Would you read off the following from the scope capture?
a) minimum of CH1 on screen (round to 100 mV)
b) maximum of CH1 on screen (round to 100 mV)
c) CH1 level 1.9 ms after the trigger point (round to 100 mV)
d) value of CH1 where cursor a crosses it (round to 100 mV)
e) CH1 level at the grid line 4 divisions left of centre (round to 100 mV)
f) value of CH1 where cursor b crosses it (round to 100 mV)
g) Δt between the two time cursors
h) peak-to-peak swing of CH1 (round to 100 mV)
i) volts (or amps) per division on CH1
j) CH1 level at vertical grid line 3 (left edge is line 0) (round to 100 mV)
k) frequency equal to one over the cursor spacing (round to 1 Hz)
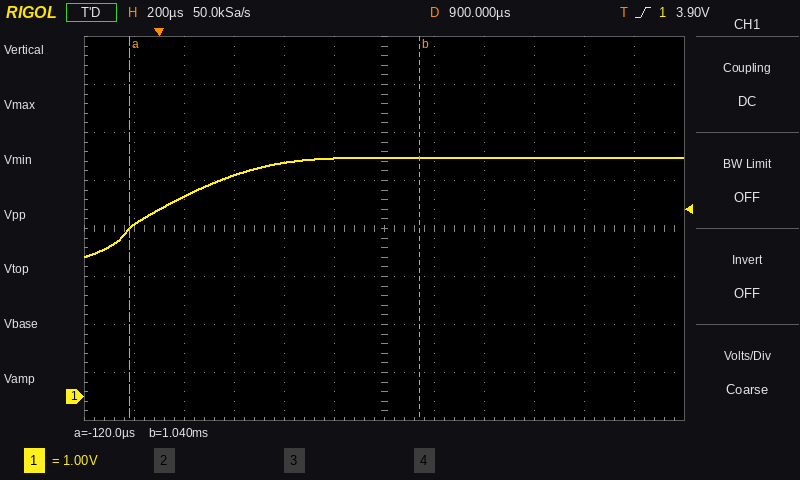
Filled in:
2.9 V
5.0 V
5.0 V
3.5 V
4.2 V
5.0 V
1.16 ms
2.1 V
1 V
4.6 V
862 Hz
